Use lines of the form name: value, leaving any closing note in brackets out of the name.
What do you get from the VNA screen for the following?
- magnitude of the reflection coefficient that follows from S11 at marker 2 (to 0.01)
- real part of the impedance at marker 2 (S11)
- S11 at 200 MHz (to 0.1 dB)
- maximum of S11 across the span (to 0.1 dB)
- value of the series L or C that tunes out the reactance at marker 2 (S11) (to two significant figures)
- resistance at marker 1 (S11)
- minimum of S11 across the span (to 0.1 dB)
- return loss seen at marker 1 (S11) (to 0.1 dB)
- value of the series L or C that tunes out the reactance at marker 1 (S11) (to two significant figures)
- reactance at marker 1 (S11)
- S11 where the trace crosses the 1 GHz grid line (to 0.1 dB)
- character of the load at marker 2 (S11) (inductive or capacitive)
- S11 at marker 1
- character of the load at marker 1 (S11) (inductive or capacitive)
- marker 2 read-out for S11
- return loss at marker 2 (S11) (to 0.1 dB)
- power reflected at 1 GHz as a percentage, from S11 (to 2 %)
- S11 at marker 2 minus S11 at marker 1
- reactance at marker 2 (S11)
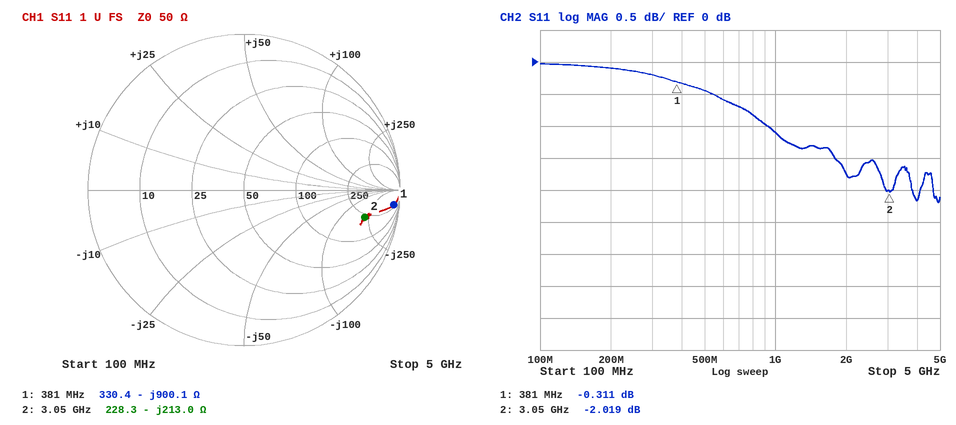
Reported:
magnitude of the reflection coefficient that follows from S11 at marker 2: 0.79
real part of the impedance at marker 2: 228.3 Ω
S11 at 200 MHz: -0.1 dB
maximum of S11 across the span: 0.0 dB
value of the series L or C that tunes out the reactance at marker 2 (S11): 11 nH
resistance at marker 1: 330.4 Ω
minimum of S11 across the span: -2.2 dB
return loss seen at marker 1 (S11): 0.3 dB
value of the series L or C that tunes out the reactance at marker 1 (S11): 380 nH
reactance at marker 1: -900.1 Ω
S11 where the trace crosses the 1 GHz grid line: -1.1 dB
character of the load at marker 2 (S11): capacitive
S11 at marker 1: -0.311 dB
character of the load at marker 1 (S11): capacitive
marker 2 read-out for S11: -2.019 dB
return loss at marker 2 (S11): 2.0 dB
power reflected at 1 GHz as a percentage, from S11: 78 %
S11 at marker 2 minus S11 at marker 1: -1.708 dB
reactance at marker 2: -213.0 Ω
